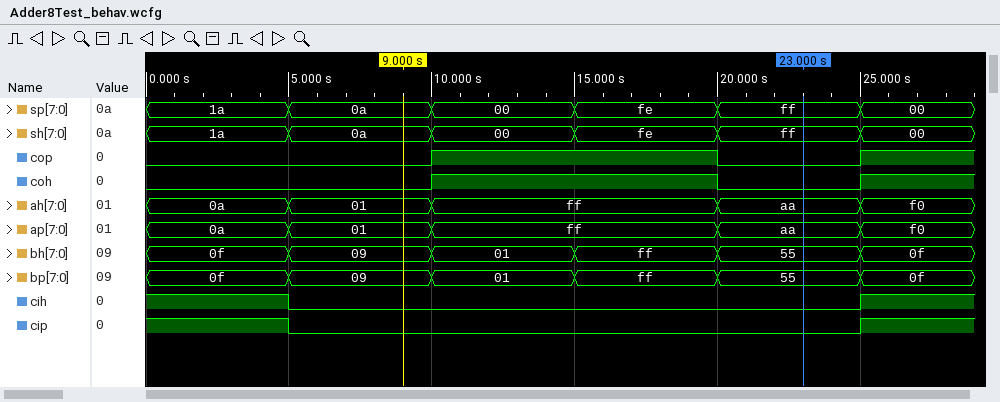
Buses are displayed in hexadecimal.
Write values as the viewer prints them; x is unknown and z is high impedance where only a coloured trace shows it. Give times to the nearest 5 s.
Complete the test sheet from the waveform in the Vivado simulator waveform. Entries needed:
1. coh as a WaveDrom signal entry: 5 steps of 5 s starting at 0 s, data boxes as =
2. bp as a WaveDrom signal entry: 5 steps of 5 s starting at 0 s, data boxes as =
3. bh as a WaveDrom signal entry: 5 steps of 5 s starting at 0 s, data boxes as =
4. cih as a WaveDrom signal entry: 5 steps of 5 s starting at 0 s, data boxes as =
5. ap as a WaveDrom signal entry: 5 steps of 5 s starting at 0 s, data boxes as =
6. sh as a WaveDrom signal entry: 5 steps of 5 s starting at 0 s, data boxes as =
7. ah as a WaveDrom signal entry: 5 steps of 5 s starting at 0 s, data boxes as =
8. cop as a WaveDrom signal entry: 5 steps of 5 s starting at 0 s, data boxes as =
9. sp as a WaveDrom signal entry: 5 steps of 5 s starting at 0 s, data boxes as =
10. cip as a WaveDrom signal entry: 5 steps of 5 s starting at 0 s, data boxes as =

{name: 'coh', wave: '0.1.0'}
{name: 'bp', wave: '=====', data: '0f 09 01 ff 55'}
{name: 'bh', wave: '=====', data: '0f 09 01 ff 55'}
{name: 'cih', wave: '10...'}
{name: 'ap', wave: '===.=', data: '0a 01 ff aa'}
{name: 'sh', wave: '=====', data: '1a 0a 00 fe ff'}
{name: 'ah', wave: '===.=', data: '0a 01 ff aa'}
{name: 'cop', wave: '0.1.0'}
{name: 'sp', wave: '=====', data: '1a 0a 00 fe ff'}
{name: 'cip', wave: '10...'}
